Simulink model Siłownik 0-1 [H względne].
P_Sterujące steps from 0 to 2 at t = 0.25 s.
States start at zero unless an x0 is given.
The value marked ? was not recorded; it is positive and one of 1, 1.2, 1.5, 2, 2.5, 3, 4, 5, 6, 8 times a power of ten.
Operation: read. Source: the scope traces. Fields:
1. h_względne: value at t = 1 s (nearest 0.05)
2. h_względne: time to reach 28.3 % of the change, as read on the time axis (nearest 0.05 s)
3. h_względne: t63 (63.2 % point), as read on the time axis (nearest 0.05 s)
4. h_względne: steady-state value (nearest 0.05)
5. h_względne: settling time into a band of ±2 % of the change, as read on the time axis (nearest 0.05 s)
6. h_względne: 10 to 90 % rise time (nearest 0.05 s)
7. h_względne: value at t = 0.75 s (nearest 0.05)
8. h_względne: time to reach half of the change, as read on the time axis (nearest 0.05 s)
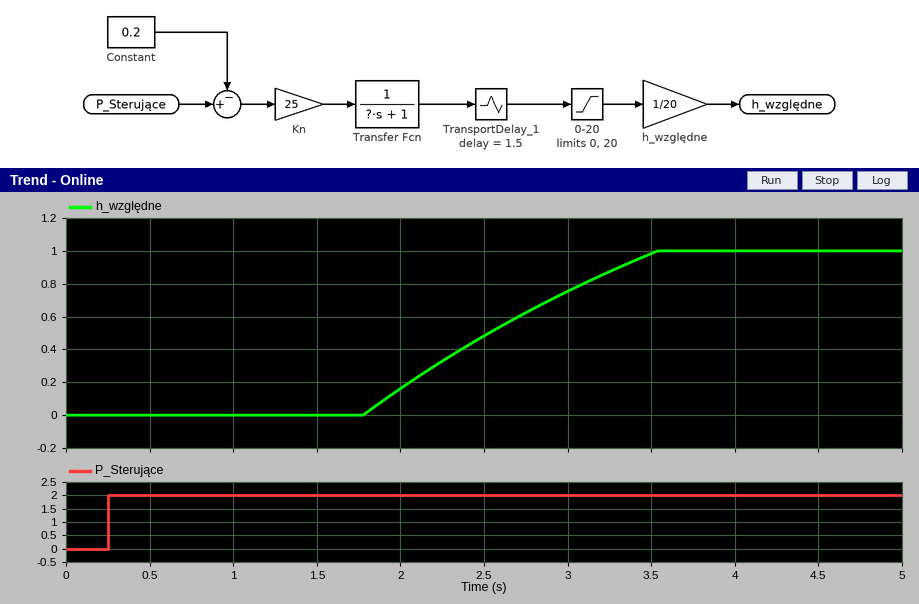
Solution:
0.00
2.20 s
2.75 s
1.00
3.50 s
1.40 s
0.00
2.55 s
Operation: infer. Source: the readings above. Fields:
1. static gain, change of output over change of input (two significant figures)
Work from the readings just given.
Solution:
0.50
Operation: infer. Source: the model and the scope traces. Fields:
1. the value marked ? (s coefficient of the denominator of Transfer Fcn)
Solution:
3
